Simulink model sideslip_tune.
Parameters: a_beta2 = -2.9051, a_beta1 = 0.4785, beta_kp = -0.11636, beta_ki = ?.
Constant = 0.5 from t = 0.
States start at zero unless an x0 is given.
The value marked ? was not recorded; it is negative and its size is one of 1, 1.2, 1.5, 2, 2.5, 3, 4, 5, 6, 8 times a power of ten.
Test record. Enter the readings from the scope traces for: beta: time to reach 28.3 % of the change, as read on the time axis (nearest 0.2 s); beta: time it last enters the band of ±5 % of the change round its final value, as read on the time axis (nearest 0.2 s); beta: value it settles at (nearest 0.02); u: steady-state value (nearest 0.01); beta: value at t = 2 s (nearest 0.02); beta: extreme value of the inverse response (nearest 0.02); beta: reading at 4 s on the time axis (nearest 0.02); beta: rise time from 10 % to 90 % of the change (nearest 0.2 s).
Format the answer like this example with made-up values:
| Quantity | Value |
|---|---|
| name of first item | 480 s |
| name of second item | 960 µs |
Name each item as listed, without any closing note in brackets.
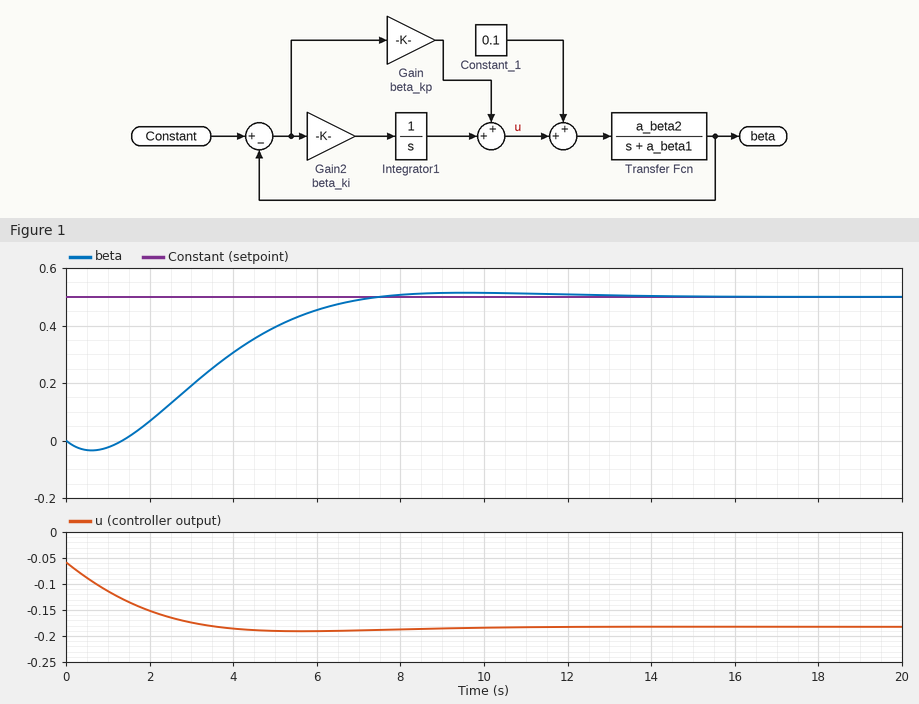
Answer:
| Quantity | Value |
|---|---|
| beta: time to reach 28.3 % of the change, as read on the time axis | 2.6 s |
| beta: time it last enters the band of ±5 % of the change round its final value, as read on the time axis | 6.6 s |
| beta: value it settles at | 0.50 |
| u: steady-state value | -0.18 |
| beta: value at t = 2 s | 0.06 |
| beta: extreme value of the inverse response | -0.04 |
| beta: reading at 4 s on the time axis | 0.30 |
| beta: rise time from 10 % to 90 % of the change | 4.0 s |
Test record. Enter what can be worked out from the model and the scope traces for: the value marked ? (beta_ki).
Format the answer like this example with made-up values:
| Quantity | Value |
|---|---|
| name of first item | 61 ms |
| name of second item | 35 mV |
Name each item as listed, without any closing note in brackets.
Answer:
| Quantity | Value |
|---|---|
| the value marked ? | -0.1 |
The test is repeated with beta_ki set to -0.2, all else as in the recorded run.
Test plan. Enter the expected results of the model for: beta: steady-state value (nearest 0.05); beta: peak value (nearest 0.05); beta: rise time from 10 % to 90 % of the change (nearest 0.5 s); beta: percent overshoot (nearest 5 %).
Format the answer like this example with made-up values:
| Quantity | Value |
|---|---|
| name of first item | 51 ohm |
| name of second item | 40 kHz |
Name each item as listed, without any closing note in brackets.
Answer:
| Quantity | Value |
|---|---|
| beta: steady-state value | 0.50 |
| beta: peak value | 0.55 |
| beta: rise time from 10 % to 90 % of the change | 2.0 s |
| beta: percent overshoot | 15 % |
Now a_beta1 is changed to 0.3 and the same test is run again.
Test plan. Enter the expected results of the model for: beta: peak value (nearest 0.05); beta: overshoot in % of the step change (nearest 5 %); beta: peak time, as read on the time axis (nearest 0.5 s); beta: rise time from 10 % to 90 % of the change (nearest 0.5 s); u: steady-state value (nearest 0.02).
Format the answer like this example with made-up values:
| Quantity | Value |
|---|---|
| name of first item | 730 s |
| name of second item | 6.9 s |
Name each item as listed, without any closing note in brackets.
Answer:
| Quantity | Value |
|---|---|
| beta: peak value | 0.55 |
| beta: overshoot in % of the step change | 10 % |
| beta: peak time, as read on the time axis | 8.0 s |
| beta: rise time from 10 % to 90 % of the change | 3.0 s |
| u: steady-state value | -0.16 |
